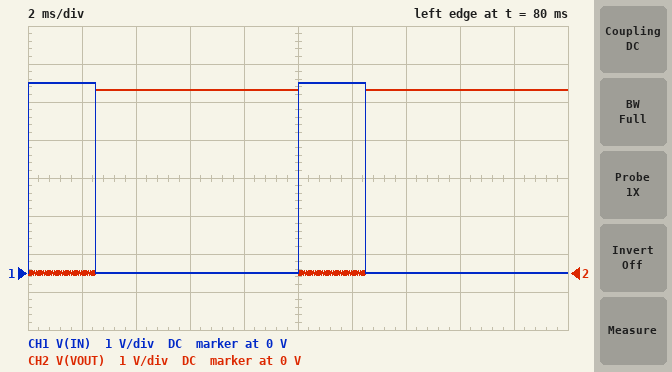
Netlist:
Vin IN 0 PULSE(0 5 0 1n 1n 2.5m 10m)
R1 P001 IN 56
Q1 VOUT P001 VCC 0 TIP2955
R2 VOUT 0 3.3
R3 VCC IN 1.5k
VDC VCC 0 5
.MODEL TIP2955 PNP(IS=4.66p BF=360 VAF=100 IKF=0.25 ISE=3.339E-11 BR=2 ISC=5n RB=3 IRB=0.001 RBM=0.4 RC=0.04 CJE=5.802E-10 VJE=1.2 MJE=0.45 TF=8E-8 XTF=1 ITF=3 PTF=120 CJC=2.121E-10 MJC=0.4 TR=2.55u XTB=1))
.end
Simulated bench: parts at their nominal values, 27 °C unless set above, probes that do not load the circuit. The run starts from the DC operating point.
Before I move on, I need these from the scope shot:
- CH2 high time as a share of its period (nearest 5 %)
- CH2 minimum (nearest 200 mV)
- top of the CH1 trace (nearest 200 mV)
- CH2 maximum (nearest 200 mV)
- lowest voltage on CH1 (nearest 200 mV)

75 %
0 V
5.0 V
4.8 V
0 V
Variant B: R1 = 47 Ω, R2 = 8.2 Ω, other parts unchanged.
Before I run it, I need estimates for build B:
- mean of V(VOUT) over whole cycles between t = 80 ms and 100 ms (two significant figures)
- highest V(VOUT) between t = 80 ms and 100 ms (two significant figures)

3.7 V
4.9 V
